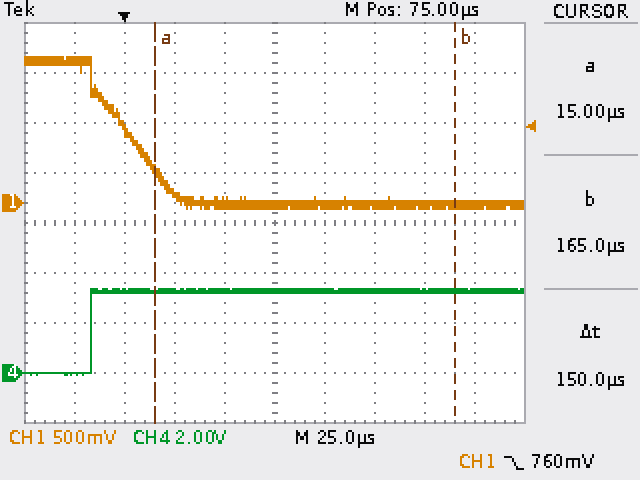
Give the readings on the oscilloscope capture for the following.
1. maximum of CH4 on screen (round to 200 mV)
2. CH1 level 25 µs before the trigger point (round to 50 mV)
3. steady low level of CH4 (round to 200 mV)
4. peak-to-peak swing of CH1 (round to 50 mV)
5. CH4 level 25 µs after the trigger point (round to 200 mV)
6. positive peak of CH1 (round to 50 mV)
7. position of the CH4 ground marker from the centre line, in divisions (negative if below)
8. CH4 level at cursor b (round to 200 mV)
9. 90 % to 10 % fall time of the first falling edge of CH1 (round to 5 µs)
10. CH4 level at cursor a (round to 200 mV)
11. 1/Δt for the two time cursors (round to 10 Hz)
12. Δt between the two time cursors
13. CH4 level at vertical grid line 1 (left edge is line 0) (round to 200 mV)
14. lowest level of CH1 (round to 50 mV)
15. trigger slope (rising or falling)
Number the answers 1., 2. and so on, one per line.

1. 3.4 V
2. 1.40 V
3. 0.0 V
4. 1.50 V
5. 3.2 V
6. 1.45 V
7. -3.0 div
8. 3.2 V
9. 40 µs
10. 3.2 V
11. 6.67 kHz
12. 150 µs
13. 0.0 V
14. -50 mV
15. falling
